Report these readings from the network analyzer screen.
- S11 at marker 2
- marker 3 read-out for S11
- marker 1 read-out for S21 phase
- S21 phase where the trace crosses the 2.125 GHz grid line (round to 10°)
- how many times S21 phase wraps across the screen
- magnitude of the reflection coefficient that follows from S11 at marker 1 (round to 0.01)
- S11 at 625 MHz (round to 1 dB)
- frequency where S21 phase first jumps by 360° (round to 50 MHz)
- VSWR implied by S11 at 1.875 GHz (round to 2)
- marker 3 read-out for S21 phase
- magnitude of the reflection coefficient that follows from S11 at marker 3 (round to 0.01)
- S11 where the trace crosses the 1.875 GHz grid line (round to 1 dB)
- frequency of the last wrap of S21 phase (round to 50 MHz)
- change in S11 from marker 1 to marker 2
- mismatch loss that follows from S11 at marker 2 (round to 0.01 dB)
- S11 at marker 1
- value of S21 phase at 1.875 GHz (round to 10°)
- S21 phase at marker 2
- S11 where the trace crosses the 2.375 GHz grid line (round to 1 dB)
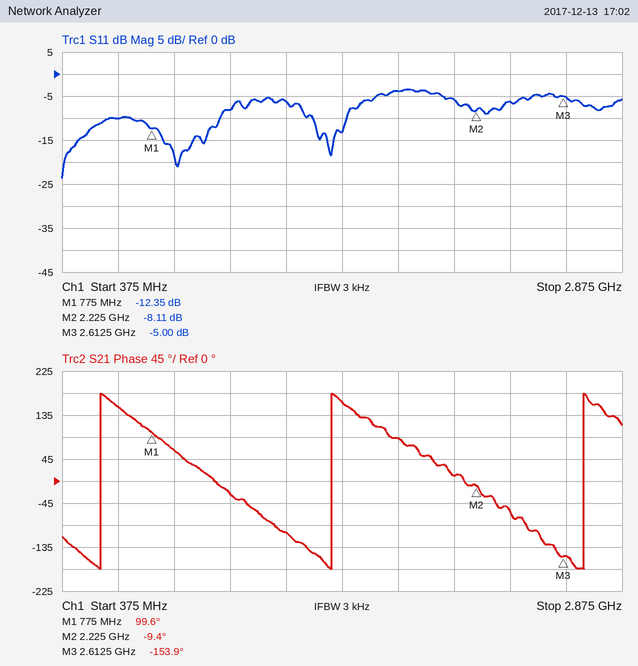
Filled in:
-8.11 dB
-5.00 dB
99.6°
10°
3
0.24
-10 dB
550 MHz
4
-153.9°
0.56
-4 dB
2.70 GHz
4.24 dB
0.73 dB
-12.35 dB
90°
-9.4°
-6 dB
